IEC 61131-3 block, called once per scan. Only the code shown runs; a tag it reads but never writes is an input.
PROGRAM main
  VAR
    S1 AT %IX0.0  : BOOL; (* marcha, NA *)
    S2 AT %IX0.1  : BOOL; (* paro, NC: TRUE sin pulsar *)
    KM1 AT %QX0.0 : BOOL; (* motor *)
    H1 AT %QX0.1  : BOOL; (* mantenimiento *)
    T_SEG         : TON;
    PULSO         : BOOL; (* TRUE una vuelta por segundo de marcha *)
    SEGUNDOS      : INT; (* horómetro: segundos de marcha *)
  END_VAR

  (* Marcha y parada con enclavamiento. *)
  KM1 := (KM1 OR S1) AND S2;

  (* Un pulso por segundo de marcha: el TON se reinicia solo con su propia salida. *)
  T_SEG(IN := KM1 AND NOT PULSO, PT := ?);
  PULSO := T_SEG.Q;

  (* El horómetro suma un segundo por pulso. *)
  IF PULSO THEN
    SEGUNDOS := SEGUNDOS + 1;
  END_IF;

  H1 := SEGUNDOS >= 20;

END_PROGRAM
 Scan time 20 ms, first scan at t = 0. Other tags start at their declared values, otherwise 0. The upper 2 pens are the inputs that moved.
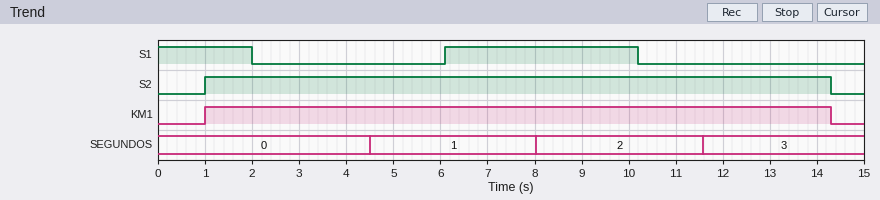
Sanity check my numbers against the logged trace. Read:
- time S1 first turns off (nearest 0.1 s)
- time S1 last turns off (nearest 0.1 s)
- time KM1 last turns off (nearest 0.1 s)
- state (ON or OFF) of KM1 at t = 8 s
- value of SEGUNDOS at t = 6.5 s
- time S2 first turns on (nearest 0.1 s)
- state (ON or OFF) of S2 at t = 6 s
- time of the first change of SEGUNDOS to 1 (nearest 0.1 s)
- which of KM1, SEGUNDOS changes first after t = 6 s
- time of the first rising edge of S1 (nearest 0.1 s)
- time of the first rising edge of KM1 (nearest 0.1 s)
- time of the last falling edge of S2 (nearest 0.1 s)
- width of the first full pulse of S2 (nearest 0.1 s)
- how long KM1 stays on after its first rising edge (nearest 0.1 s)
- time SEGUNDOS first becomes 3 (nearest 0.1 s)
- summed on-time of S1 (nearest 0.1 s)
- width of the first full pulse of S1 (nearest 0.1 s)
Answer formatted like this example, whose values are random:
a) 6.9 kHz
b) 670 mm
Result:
a) 2.0 s
b) 10.2 s
c) 14.3 s
d) ON
e) 1
f) 1.0 s
g) ON
h) 4.5 s
i) SEGUNDOS
j) 6.1 s
k) 1.0 s
l) 14.3 s
m) 13.3 s
n) 13.3 s
o) 11.6 s
p) 6.1 s
q) 4.1 s
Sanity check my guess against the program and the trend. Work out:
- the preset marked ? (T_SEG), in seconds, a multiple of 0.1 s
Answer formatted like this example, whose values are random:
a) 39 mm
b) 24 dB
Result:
a) 3.5 s
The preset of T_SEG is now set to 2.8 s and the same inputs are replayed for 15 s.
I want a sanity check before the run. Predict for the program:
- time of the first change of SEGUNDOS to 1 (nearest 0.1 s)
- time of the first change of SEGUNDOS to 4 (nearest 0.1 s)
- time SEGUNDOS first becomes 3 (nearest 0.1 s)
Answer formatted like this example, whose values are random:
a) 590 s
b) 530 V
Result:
a) 3.8 s
b) 12.3 s
c) 9.5 s
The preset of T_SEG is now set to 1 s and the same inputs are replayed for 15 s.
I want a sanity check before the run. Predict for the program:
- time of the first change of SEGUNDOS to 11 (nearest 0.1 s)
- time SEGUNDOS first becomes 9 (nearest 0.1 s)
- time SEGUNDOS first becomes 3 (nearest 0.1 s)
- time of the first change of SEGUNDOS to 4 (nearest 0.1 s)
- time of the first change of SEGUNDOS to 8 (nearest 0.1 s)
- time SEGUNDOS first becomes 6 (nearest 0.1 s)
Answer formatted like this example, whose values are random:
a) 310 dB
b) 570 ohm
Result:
a) 12.4 s
b) 10.3 s
c) 4.1 s
d) 5.1 s
e) 9.3 s
f) 7.2 s
